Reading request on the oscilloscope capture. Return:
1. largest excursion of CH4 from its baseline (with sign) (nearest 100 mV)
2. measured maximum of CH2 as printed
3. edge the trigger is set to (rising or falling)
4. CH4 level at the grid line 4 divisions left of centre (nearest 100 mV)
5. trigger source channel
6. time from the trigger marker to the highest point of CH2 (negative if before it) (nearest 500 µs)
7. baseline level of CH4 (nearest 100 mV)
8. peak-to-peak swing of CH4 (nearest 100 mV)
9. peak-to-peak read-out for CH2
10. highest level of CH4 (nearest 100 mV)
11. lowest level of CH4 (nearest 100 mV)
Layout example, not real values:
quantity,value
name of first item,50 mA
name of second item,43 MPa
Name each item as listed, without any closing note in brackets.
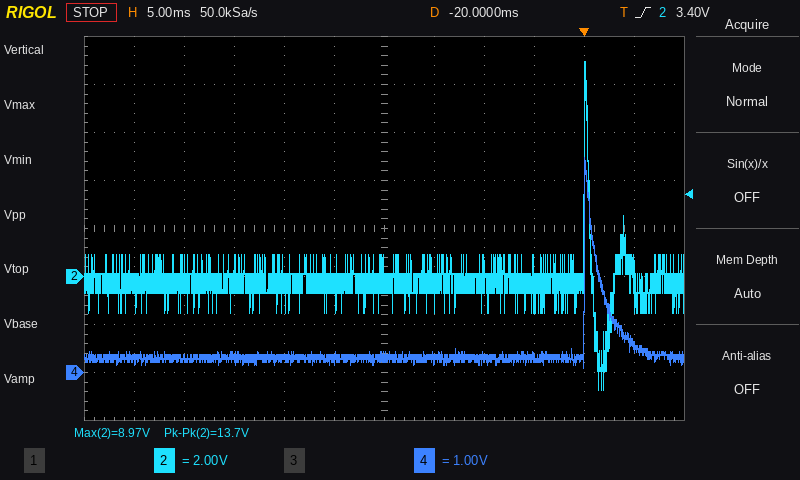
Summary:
quantity,value
largest excursion of CH4 from its baseline (with sign),+4.2 V
measured maximum of CH2 as printed,8.97 V
edge the trigger is set to,rising
CH4 level at the grid line 4 divisions left of centre,300 mV
trigger source channel,CH2
time from the trigger marker to the highest point of CH2 (negative if before it),0.0 ms
baseline level of CH4,300 mV
peak-to-peak swing of CH4,4.4 V
peak-to-peak read-out for CH2,13.7 V
highest level of CH4,4.5 V
lowest level of CH4,100 mV
